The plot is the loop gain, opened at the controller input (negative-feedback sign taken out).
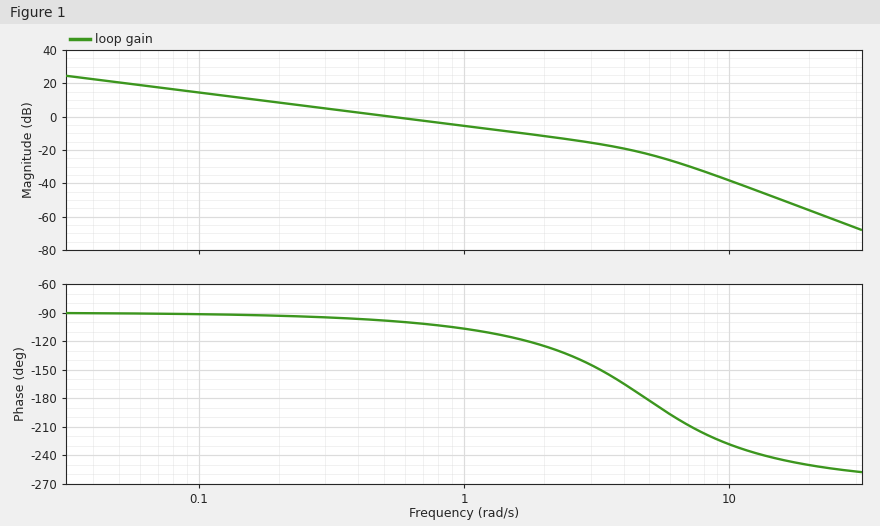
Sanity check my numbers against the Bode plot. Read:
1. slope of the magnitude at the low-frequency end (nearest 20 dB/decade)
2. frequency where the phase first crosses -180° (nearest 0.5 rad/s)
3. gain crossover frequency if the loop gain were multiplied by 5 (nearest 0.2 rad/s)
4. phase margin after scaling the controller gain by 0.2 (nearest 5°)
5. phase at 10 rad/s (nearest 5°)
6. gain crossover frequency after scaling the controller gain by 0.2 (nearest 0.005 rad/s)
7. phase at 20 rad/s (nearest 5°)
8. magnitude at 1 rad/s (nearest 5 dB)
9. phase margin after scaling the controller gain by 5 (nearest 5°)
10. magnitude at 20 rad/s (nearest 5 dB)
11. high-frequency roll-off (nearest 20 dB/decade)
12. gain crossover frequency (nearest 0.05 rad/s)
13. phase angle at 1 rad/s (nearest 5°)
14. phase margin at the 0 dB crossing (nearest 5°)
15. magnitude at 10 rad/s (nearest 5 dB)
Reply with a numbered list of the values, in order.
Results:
1. -20 dB/decade
2. 5.0 rad/s
3. 2.6 rad/s
4. 90°
5. -230°
6. 0.105 rad/s
7. -250°
8. -5 dB
9. 45°
10. -55 dB
11. -60 dB/decade
12. 0.55 rad/s
13. -105°
14. 80°
15. -40 dB
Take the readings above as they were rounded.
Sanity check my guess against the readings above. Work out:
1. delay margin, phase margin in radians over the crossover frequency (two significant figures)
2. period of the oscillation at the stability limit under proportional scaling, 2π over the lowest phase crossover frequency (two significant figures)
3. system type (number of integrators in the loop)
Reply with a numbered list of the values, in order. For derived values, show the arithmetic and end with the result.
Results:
1. 80 × π / 180 / 0.55 = 2.5 s
2. 2π / 5 = 1.3 s
3. 1
